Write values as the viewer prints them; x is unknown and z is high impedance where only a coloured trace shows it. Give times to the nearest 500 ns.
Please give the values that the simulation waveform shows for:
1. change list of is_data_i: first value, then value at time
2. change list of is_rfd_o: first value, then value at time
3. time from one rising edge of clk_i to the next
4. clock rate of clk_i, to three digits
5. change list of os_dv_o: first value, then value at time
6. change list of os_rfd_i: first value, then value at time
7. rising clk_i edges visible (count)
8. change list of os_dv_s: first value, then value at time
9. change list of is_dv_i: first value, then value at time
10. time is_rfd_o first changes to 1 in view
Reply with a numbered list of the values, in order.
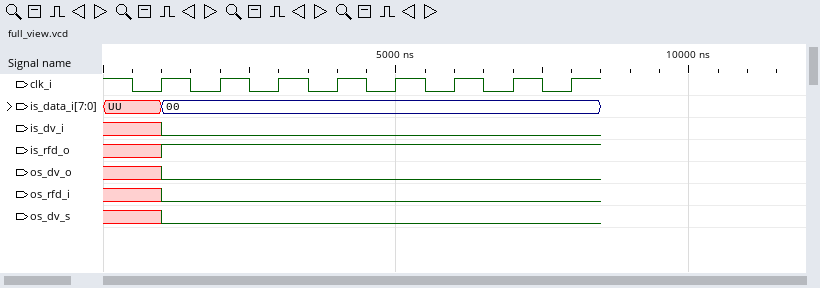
1. UU, 00 at 1000 ns
2. x, 1 at 1000 ns
3. 1000 ns
4. 1.00 MHz
5. x, 0 at 1000 ns
6. x, 0 at 1000 ns
7. 8
8. x, 0 at 1000 ns
9. x, 0 at 1000 ns
10. 1000 ns
